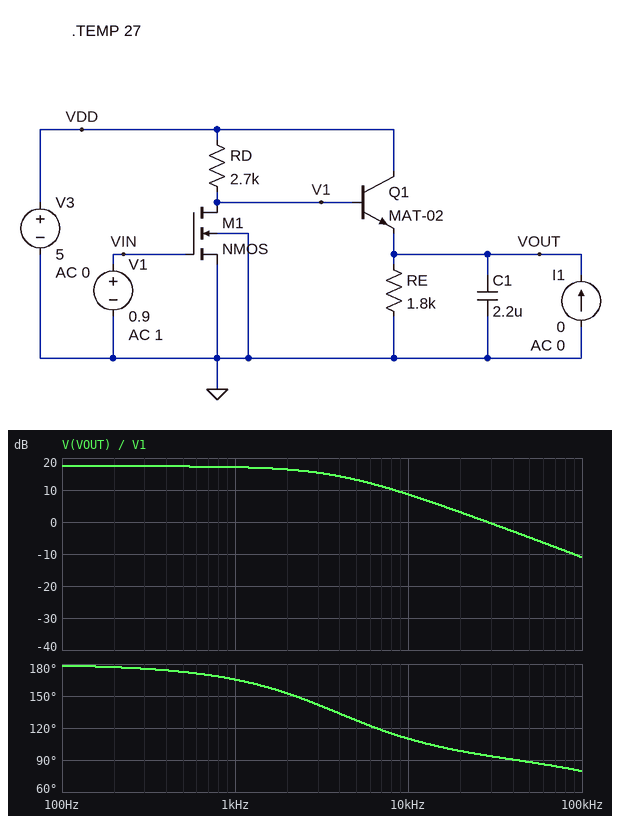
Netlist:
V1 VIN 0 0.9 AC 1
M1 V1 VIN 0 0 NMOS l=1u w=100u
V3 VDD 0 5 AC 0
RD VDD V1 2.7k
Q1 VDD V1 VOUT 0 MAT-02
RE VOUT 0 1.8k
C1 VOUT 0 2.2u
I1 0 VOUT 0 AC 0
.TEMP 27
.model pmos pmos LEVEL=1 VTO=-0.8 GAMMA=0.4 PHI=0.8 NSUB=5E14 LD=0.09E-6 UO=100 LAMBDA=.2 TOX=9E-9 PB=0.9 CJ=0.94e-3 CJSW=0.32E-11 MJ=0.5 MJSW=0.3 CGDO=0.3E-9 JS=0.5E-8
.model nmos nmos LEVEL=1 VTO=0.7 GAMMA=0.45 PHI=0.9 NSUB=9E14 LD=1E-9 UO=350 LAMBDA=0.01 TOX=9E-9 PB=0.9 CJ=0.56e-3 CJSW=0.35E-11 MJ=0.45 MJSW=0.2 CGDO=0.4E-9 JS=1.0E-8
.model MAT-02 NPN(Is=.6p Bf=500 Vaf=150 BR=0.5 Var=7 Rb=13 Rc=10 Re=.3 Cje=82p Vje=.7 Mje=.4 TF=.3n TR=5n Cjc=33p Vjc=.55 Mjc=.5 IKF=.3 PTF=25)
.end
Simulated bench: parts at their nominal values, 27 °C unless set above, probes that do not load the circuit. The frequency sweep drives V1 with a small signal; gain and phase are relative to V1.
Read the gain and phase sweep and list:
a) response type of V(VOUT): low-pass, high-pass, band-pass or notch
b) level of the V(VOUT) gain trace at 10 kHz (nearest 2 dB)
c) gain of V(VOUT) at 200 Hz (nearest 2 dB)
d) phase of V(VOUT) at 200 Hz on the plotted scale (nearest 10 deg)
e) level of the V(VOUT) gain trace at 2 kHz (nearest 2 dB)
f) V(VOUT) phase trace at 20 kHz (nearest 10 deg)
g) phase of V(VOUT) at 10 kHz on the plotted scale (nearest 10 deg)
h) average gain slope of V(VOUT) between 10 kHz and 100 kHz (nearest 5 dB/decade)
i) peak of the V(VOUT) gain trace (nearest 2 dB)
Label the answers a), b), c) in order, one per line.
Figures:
a) low-pass
b) 8 dB
c) 18 dB
d) 180 deg
e) 16 dB
f) 100 deg
g) 110 deg
h) -20 dB/decade
i) 18 dB
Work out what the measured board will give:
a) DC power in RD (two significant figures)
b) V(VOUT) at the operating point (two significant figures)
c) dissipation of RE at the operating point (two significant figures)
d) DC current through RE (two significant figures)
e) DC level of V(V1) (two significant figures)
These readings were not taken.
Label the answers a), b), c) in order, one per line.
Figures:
a) 220 µW
b) 3.7 V
c) 7.4 mW
d) 2.0 mA
e) 4.2 V
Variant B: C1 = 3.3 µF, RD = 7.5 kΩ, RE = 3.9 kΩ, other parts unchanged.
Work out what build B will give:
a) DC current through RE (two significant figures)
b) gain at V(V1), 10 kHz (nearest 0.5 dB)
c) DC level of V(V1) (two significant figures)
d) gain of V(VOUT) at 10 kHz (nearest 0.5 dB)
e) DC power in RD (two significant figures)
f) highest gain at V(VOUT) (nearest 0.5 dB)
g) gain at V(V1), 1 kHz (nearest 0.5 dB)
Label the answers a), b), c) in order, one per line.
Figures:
a) 610 µA
b) 23.5 dB
c) 2.9 V
d) 4.5 dB
e) 580 µW
f) 26.0 dB
g) 25.0 dB
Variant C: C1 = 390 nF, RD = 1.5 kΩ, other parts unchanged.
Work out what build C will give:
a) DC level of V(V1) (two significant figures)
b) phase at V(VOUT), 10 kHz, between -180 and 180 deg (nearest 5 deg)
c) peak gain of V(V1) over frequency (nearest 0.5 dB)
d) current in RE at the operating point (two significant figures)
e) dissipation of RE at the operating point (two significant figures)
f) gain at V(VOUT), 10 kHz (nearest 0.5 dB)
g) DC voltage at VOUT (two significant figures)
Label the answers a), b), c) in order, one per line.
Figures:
a) 4.6 V
b) 160 deg
c) 12.5 dB
d) 2.2 mA
e) 8.9 mW
f) 12.0 dB
g) 4.0 V
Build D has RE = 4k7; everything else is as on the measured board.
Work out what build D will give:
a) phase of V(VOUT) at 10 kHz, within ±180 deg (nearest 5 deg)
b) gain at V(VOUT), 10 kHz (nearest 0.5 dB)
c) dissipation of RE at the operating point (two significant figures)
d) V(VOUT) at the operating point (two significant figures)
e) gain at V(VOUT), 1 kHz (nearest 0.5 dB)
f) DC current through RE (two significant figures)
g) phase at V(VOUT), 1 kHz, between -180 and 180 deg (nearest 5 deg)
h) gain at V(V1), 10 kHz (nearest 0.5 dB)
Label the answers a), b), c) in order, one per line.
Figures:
a) 100 deg
b) 2.5 dB
c) 2.9 mW
d) 3.7 V
e) 16.5 dB
f) 790 µA
g) 150 deg
h) 16.0 dB
